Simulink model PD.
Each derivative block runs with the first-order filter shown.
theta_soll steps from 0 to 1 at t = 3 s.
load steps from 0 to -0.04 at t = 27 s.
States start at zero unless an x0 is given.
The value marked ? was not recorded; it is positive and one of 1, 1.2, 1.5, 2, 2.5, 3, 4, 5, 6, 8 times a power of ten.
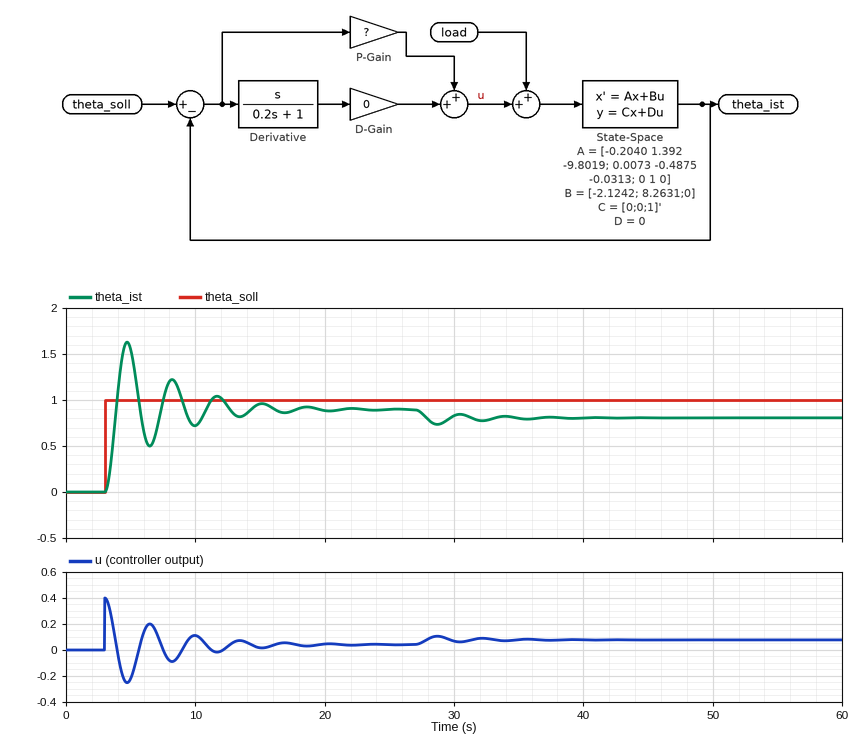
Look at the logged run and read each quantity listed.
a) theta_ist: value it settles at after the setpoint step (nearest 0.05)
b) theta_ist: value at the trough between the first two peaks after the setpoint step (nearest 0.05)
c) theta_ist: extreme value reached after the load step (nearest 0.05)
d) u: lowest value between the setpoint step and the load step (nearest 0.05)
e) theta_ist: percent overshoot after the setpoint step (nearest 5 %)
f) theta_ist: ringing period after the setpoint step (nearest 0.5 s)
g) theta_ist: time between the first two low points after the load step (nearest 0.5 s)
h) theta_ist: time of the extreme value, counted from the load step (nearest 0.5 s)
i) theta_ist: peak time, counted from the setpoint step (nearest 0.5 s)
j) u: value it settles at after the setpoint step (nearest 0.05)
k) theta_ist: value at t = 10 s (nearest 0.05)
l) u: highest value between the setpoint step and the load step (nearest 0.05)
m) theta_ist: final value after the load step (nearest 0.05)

0.90
0.50
0.75
-0.25
80 %
3.5 s
3.5 s
1.5 s
1.5 s
0.05
0.70
0.40
0.80
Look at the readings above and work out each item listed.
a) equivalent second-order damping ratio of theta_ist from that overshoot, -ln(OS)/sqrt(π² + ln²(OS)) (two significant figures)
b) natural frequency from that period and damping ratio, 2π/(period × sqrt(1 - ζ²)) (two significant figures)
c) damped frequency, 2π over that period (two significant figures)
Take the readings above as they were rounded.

0.071
1.8 rad/s
1.8 rad/s
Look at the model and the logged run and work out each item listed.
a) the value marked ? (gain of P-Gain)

0.4
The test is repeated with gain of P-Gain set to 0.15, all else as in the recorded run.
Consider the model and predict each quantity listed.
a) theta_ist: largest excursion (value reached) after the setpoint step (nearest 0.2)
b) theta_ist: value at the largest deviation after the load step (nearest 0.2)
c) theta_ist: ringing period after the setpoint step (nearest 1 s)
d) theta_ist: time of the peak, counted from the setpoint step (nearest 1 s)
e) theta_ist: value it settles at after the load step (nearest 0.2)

1.4
0.4
6 s
3 s
0.6
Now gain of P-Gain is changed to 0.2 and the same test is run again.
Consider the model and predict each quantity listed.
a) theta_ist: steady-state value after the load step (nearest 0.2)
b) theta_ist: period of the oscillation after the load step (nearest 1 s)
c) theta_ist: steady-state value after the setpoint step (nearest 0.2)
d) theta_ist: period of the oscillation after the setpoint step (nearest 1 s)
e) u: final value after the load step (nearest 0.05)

0.6
5 s
0.8
5 s
0.05
